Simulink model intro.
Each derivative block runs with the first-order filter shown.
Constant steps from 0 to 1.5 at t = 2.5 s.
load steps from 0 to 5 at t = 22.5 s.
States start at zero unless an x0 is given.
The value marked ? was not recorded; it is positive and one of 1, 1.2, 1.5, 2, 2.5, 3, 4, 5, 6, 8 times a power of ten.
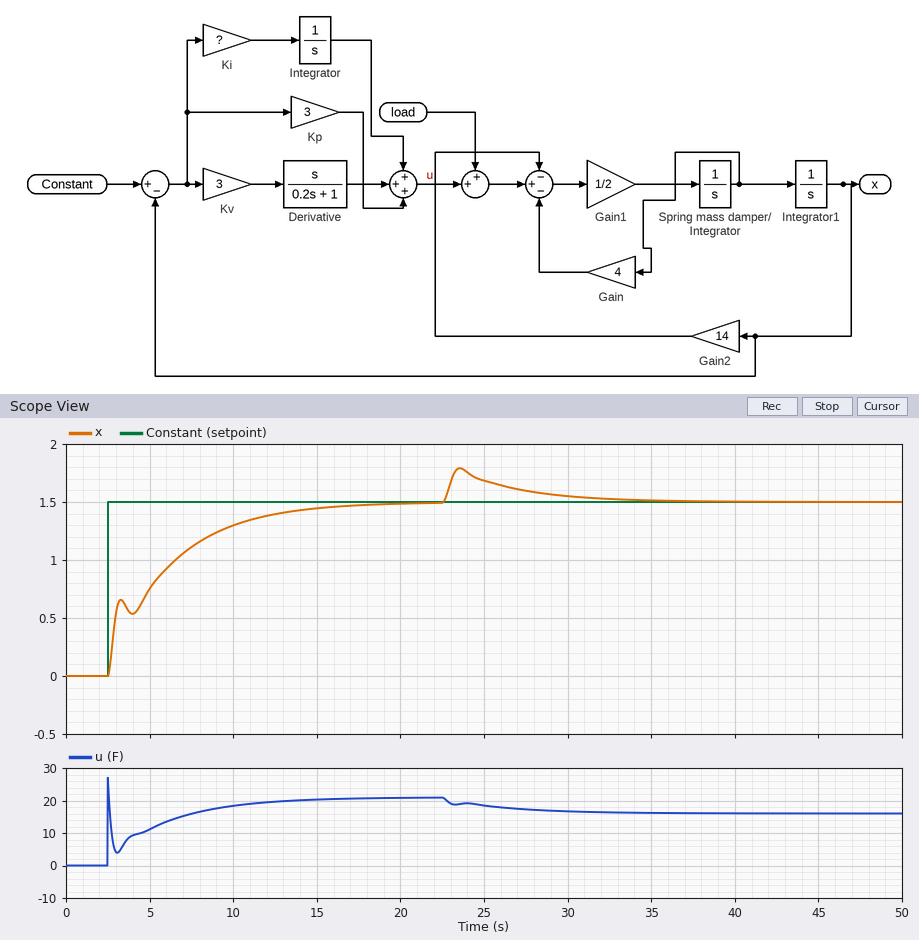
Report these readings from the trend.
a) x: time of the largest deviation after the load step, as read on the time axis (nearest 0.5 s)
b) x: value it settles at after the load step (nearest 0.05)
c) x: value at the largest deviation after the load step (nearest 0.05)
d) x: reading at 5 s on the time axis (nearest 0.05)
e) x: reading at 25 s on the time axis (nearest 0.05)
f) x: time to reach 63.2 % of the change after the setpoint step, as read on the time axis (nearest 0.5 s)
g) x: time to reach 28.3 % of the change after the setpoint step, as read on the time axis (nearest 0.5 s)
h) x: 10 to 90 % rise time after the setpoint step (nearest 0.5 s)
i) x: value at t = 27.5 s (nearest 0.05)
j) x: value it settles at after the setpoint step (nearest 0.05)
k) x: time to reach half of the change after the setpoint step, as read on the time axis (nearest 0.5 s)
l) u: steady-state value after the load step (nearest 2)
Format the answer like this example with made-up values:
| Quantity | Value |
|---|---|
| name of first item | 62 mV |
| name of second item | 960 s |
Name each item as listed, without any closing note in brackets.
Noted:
| Quantity | Value |
|---|---|
| x: time of the largest deviation after the load step, as read on the time axis | 23.5 s |
| x: value it settles at after the load step | 1.50 |
| x: value at the largest deviation after the load step | 1.80 |
| x: reading at 5 s on the time axis | 0.75 |
| x: reading at 25 s on the time axis | 1.70 |
| x: time to reach 63.2 % of the change after the setpoint step, as read on the time axis | 6.0 s |
| x: time to reach 28.3 % of the change after the setpoint step, as read on the time axis | 3.0 s |
| x: 10 to 90 % rise time after the setpoint step | 8.5 s |
| x: value at t = 27.5 s | 1.60 |
| x: value it settles at after the setpoint step | 1.50 |
| x: time to reach half of the change after the setpoint step, as read on the time axis | 5.0 s |
| u: steady-state value after the load step | 16 |
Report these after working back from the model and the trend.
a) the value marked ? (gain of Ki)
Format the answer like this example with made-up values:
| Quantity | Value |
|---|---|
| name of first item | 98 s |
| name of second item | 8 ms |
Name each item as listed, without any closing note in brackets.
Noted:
| Quantity | Value |
|---|---|
| the value marked ? | 4 |
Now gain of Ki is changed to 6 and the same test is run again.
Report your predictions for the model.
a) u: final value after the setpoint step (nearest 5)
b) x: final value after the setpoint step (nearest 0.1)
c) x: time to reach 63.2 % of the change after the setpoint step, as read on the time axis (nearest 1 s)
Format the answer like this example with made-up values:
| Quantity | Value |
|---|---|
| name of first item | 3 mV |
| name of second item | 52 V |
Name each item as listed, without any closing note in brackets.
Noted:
| Quantity | Value |
|---|---|
| u: final value after the setpoint step | 20 |
| x: final value after the setpoint step | 1.5 |
| x: time to reach 63.2 % of the change after the setpoint step, as read on the time axis | 5 s |
